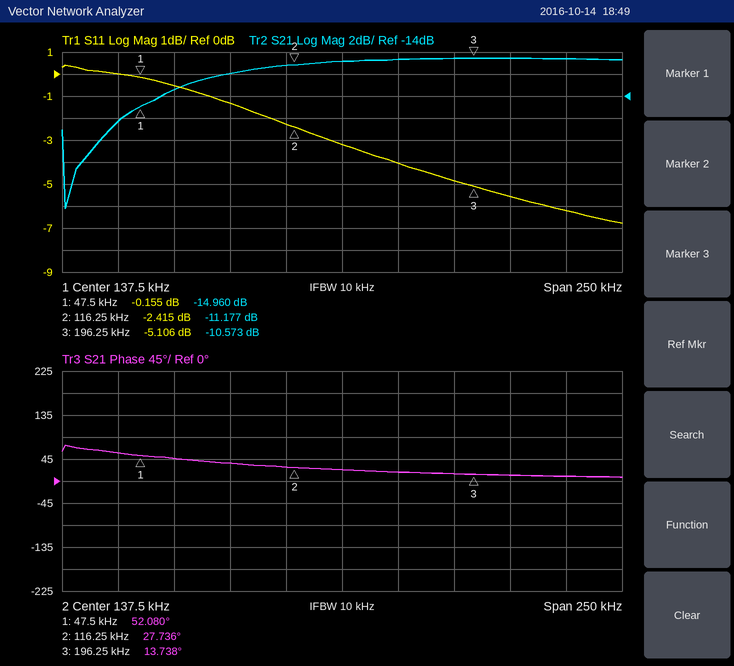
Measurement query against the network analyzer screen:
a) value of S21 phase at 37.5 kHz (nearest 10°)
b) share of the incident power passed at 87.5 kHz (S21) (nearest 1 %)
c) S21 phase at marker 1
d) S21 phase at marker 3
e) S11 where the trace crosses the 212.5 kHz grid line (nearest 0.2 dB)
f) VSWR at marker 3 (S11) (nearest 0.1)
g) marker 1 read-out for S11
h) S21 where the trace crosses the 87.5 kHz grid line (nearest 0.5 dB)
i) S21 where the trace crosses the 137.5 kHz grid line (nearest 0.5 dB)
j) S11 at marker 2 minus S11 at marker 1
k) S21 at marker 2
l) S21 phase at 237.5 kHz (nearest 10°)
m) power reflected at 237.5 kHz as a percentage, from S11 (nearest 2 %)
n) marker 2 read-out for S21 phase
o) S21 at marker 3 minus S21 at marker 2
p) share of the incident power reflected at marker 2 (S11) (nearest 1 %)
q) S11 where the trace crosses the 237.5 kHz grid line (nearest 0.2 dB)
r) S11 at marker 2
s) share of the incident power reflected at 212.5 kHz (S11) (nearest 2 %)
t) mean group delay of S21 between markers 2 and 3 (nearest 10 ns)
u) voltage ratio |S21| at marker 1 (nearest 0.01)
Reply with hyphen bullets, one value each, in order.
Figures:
- 60°
- 6 %
- 52.080°
- 13.738°
- -5.6 dB
- 3.5
- -0.155 dB
- -12.0 dB
- -11.0 dB
- -2.260 dB
- -11.177 dB
- 10°
- 24 %
- 27.736°
- 0.604 dB
- 57 %
- -6.2 dB
- -2.415 dB
- 28 %
- 490 ns
- 0.18
